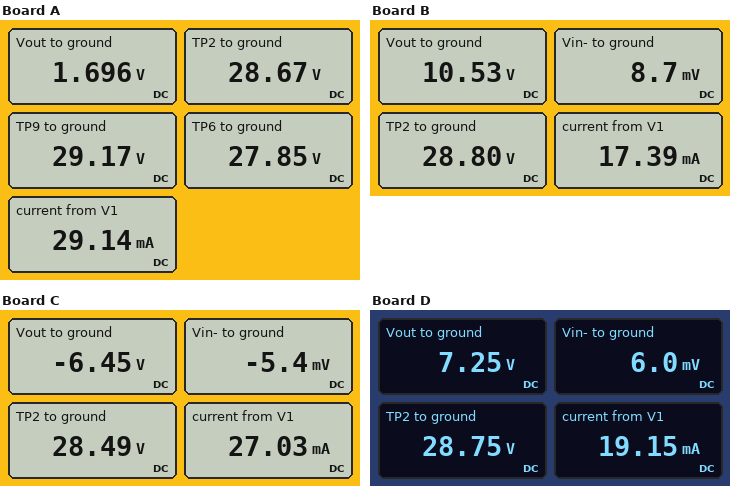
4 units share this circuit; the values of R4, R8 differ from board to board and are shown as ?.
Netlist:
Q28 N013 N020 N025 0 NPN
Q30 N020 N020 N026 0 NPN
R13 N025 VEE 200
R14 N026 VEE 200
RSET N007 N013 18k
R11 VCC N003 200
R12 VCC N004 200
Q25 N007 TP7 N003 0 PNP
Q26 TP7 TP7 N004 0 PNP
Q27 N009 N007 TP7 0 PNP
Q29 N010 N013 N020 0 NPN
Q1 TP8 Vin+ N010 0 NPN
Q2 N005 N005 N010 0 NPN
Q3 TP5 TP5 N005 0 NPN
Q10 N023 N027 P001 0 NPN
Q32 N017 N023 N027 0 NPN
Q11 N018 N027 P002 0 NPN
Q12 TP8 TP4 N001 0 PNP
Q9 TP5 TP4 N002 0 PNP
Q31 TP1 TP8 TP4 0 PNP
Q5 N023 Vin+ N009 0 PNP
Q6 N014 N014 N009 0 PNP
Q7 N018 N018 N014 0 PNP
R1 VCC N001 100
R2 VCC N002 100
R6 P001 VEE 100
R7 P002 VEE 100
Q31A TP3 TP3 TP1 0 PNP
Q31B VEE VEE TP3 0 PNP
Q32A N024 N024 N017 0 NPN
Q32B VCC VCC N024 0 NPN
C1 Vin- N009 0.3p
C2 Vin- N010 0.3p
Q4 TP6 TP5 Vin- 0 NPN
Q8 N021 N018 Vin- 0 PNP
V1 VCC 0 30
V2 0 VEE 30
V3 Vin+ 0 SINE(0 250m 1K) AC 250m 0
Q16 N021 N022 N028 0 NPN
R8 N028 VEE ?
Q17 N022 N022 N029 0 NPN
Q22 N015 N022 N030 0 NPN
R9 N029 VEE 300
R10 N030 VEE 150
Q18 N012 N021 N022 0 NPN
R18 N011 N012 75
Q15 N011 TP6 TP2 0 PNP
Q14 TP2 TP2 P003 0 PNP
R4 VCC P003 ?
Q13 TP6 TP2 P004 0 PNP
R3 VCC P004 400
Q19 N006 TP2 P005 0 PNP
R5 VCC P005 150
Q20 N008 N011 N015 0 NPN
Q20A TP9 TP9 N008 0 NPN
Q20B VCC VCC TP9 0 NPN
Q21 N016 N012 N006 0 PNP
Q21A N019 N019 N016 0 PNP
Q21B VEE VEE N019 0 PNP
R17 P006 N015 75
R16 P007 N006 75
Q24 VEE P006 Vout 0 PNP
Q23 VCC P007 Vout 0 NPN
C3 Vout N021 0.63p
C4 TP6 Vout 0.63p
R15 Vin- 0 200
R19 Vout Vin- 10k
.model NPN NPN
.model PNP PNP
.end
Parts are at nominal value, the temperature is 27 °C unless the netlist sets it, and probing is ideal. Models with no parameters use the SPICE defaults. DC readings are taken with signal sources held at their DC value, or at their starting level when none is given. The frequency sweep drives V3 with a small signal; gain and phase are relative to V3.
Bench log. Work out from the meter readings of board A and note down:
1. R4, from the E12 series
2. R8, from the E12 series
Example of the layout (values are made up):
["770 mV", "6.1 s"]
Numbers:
["100 Ω", "1 kΩ"]
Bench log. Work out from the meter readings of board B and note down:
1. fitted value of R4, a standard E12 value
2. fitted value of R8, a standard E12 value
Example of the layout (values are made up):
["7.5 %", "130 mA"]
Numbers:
["390 Ω", "150 Ω"]
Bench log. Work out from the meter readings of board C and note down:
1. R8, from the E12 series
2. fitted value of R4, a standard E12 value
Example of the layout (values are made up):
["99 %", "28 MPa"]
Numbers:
["1 kΩ", "180 Ω"]
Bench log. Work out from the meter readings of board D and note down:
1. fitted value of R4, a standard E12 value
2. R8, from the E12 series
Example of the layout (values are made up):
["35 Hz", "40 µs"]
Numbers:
["270 Ω", "270 Ω"]
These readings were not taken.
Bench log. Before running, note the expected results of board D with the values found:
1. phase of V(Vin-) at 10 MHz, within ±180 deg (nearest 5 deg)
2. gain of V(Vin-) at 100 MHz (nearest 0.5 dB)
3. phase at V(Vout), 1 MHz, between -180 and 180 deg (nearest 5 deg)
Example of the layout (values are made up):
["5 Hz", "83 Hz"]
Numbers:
["0 deg", "-0.5 dB", "-5 deg"]
